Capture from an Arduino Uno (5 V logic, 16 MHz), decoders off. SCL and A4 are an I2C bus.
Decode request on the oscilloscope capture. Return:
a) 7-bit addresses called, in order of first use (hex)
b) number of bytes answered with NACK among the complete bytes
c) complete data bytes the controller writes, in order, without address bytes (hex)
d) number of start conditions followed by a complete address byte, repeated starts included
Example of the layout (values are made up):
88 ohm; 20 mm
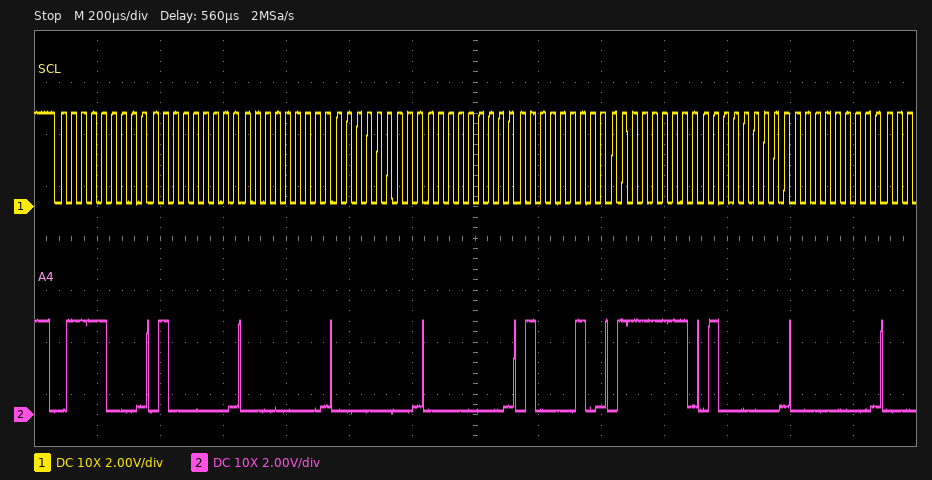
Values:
0x3C; 0; 40 00 00 00 42 7F 40 00; 1
